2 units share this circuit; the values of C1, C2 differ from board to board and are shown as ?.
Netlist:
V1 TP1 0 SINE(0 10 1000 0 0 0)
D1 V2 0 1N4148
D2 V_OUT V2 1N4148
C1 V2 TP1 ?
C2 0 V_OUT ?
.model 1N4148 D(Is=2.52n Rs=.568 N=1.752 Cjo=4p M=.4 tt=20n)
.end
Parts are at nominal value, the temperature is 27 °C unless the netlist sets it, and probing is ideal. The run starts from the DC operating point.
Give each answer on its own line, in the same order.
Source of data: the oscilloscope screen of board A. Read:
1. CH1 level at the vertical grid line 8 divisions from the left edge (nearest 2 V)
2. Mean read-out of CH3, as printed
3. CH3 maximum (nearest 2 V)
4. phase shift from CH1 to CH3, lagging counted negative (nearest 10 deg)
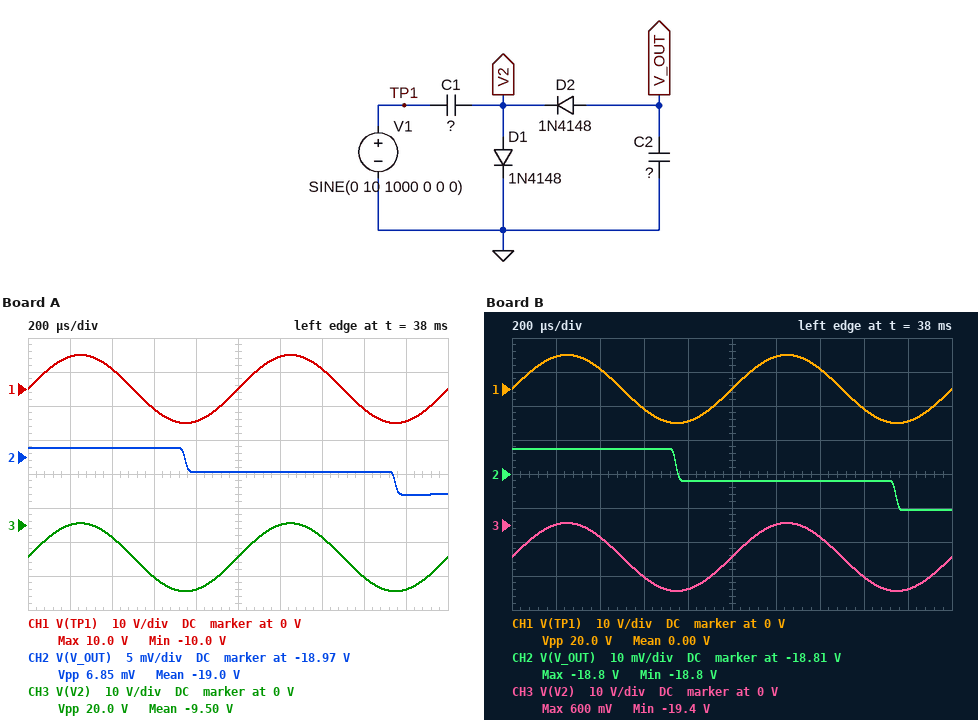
-6 V
-9.50 V
0 V
0 deg
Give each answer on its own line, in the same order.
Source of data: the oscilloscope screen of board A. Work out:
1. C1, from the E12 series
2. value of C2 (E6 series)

680 nF
1.5 µF
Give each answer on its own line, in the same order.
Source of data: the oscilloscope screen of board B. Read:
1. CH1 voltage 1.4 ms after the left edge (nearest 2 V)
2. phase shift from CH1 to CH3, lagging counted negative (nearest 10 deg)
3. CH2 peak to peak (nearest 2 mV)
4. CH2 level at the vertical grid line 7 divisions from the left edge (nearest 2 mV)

6 V
0 deg
18 mV
-18.812 V
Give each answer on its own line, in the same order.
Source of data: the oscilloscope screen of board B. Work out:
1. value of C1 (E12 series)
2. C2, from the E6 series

560 nF
3.3 µF
